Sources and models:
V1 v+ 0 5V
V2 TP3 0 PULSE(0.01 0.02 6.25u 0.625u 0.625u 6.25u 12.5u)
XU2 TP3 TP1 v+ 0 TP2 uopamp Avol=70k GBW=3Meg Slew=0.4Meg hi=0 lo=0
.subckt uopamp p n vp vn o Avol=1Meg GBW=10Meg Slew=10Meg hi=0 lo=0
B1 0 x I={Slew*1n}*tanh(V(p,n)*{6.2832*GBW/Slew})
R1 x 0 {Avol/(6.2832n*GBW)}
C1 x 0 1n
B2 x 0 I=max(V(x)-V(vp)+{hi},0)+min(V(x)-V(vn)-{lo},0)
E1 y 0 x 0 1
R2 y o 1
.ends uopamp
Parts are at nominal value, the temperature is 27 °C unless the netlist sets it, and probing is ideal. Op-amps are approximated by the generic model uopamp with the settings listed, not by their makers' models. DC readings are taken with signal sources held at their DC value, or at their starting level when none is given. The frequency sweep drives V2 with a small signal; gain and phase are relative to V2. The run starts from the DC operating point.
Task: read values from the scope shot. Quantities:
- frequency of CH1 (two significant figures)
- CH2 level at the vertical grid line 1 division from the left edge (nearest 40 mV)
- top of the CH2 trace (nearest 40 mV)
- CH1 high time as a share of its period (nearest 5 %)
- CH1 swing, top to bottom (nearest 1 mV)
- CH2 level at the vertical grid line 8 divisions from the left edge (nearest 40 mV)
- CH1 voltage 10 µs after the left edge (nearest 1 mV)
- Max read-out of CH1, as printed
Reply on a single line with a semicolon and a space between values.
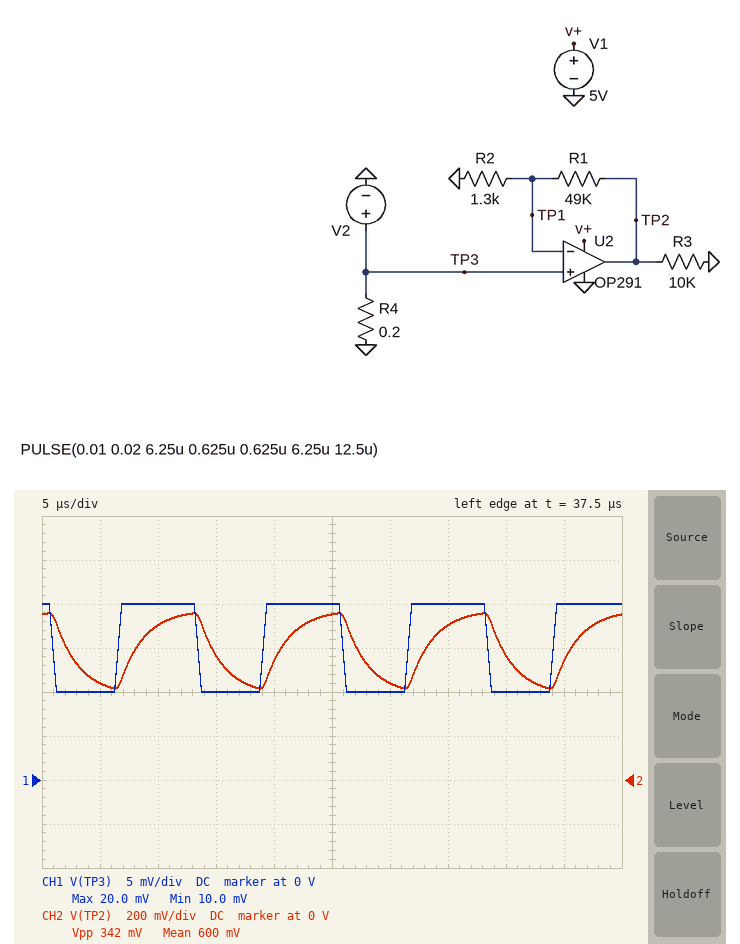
80 kHz; 440 mV; 760 mV; 55 %; 10 mV; 560 mV; 20 mV; 20.0 mV
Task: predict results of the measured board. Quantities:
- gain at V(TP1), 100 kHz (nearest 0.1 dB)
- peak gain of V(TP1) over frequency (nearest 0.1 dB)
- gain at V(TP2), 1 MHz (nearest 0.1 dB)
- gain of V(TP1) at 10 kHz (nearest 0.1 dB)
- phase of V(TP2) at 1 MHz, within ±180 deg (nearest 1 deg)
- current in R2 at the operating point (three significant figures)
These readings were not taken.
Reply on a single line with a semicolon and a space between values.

-4.3 dB; 0 dB; 9.5 dB; -0.1 dB; -86 deg; 7.69 µA
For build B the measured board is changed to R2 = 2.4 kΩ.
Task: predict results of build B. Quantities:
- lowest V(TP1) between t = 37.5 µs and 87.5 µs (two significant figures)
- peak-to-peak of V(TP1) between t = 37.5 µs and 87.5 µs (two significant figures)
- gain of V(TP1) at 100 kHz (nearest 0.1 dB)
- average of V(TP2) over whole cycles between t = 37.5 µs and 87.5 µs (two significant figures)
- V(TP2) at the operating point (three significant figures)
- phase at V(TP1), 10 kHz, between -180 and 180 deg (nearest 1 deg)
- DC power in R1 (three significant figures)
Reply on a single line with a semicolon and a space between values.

10 mV; 9.9 mV; -1.8 dB; 330 mV; 214 mV; -4 deg; 850 nW
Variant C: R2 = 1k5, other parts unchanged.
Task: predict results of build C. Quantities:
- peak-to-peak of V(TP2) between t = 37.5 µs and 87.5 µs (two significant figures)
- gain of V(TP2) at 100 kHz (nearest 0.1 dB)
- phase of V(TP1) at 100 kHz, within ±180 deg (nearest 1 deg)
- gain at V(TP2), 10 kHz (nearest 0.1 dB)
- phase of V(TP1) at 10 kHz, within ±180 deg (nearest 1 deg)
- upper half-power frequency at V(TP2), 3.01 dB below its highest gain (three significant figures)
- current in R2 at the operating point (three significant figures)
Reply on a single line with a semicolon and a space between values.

310 mV; 27.0 dB; -48 deg; 30.5 dB; -6 deg; 89.1 kHz; 6.66 µA
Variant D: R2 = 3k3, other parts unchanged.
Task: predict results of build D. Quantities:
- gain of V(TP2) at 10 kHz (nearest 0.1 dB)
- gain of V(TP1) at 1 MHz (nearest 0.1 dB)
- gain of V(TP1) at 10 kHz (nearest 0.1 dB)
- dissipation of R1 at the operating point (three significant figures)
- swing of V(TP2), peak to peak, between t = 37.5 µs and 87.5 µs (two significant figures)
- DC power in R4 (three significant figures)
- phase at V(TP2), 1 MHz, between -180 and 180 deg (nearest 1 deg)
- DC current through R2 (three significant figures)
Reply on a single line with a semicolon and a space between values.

24.0 dB; -14.6 dB; 0 dB; 450 nW; 160 mV; 500 µW; -79 deg; 3.03 µA
